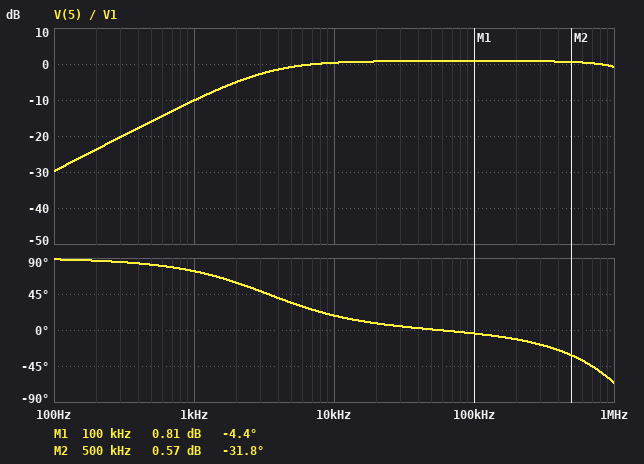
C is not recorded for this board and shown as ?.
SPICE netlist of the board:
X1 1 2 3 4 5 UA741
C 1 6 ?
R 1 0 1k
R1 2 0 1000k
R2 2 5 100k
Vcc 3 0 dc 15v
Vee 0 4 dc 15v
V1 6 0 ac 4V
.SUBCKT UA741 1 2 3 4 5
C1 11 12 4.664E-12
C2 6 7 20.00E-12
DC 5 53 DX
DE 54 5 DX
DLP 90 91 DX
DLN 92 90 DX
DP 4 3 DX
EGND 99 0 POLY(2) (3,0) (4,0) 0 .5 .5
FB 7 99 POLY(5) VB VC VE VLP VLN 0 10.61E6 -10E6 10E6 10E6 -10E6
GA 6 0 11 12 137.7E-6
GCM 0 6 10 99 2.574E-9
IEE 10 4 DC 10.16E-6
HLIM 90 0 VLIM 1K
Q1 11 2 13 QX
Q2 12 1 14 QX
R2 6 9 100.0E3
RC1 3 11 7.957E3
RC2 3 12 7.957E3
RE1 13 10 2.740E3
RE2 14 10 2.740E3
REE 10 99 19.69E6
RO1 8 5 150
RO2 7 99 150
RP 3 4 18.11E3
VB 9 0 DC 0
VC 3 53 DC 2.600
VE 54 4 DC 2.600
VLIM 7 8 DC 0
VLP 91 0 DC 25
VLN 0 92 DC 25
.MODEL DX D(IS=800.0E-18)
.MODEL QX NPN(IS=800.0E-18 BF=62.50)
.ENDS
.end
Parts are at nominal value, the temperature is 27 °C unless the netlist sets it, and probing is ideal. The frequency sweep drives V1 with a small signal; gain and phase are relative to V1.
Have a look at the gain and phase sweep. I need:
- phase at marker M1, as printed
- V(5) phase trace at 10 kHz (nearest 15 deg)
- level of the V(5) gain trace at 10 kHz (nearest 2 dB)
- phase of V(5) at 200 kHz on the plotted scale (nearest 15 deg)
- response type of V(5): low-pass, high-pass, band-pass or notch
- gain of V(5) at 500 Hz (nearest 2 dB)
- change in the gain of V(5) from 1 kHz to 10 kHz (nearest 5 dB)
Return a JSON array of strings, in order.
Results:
["-4.4 deg", "15 deg", "0 dB", "-15 deg", "high-pass", "-16 dB", "10 dB"]
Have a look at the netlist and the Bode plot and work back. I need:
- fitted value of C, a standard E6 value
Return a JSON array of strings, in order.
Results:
["47 nF"]
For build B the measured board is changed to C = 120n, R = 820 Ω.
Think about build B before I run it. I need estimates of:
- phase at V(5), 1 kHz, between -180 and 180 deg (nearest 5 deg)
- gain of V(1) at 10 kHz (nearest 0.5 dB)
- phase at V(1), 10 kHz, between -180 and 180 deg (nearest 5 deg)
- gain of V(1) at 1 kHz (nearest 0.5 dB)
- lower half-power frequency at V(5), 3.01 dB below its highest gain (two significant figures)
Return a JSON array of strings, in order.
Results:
["60 deg", "0 dB", "10 deg", "-5.5 dB", "1.6 kHz"]
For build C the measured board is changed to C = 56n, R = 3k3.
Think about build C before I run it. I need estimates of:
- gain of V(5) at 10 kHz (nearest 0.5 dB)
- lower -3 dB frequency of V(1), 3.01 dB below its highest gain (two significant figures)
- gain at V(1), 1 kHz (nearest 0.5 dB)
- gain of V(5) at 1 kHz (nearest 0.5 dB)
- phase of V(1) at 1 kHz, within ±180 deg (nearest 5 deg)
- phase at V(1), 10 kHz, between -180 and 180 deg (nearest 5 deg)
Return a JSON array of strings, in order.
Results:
["1.0 dB", "860 Hz", "-2.5 dB", "-1.5 dB", "40 deg", "5 deg"]
